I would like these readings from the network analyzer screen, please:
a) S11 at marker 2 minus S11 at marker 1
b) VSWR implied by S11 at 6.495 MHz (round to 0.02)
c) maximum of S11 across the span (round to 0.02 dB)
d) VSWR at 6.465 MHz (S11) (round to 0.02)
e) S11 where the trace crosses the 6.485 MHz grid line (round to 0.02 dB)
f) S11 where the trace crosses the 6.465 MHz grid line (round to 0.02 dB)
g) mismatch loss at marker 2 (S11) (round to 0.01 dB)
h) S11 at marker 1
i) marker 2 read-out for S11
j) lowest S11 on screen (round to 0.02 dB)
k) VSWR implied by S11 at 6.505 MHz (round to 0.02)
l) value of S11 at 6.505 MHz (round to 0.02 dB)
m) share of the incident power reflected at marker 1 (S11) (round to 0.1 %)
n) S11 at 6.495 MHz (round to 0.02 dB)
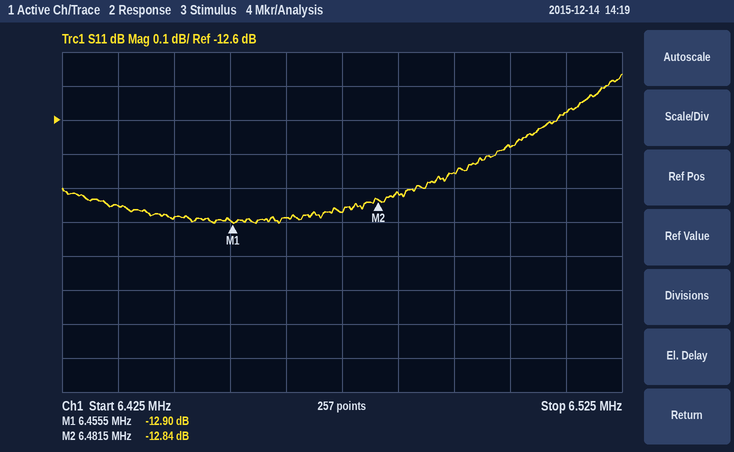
0.06 dB
1.60
-12.46 dB
1.58
-12.82 dB
-12.88 dB
0.23 dB
-12.90 dB
-12.84 dB
-12.90 dB
1.60
-12.68 dB
5.1 %
-12.76 dB
